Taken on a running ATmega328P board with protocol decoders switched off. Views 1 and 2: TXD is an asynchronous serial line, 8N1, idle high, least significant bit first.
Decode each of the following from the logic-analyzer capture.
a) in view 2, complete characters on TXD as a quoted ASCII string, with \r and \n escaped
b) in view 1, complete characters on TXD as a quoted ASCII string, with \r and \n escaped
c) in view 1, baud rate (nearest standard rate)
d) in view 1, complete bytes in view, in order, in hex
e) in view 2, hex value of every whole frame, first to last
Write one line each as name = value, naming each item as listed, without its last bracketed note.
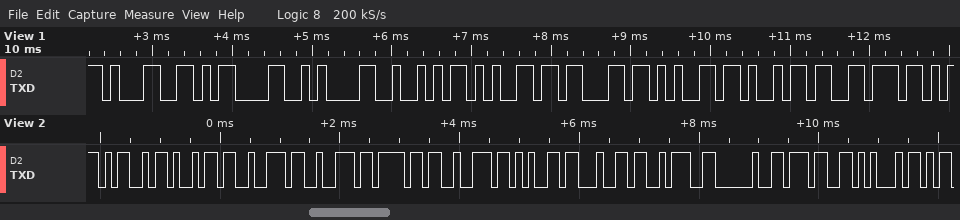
in view 2, complete characters on TXD as a quoted ASCII string, with \r and \n escaped = "Mirrored: 7E"
in view 1, complete characters on TXD as a quoted ASCII string, with \r and \n escaped = "1\r\nReceiv"
in view 1, baud rate = 9600 baud
in view 1, complete bytes in view, in order, in hex = 0x31 0x0D 0x0A 0x52 0x65 0x63 0x65 0x69 0x76
in view 2, hex value of every whole frame, first to last = 4D 69 72 72 6F 72 65 64 3A 20 37 45
